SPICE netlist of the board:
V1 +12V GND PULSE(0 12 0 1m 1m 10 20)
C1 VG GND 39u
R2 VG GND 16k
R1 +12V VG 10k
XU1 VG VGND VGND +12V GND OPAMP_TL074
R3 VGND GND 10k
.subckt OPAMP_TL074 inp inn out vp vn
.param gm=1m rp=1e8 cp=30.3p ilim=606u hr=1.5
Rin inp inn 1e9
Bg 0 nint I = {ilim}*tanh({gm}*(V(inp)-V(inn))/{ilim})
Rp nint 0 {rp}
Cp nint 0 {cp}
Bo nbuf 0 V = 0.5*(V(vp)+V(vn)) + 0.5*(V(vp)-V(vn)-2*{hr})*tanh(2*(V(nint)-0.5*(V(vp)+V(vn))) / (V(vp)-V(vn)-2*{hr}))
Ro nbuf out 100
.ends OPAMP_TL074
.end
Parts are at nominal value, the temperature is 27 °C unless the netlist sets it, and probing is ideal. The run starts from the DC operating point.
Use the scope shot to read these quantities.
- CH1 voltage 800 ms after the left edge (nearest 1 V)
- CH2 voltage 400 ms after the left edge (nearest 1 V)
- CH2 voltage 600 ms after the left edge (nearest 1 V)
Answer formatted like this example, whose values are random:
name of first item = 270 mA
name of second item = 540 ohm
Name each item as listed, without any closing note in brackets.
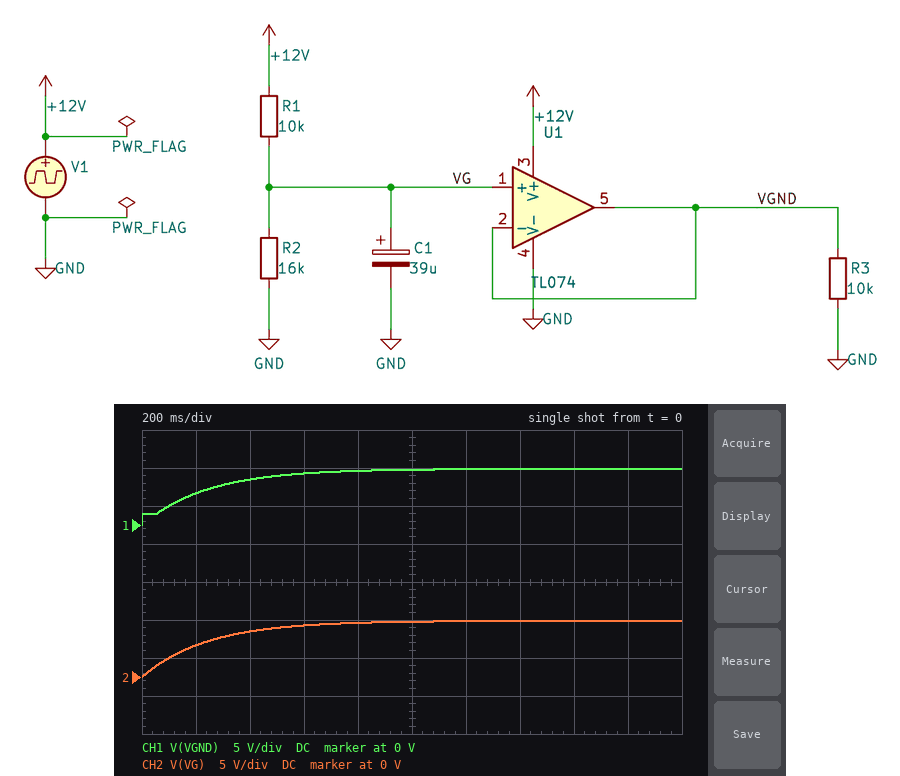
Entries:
CH1 voltage 800 ms after the left edge = 7 V
CH2 voltage 400 ms after the left edge = 6 V
CH2 voltage 600 ms after the left edge = 7 V
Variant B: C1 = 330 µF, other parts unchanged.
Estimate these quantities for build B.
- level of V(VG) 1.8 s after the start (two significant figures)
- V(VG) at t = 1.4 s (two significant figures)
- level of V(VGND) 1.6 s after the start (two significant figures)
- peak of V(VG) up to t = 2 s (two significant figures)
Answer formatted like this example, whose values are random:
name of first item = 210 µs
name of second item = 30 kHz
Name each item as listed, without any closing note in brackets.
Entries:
level of V(VG) 1.8 s after the start = 4.3 V
V(VG) at t = 1.4 s = 3.7 V
level of V(VGND) 1.6 s after the start = 4.0 V
peak of V(VG) up to t = 2 s = 4.6 V
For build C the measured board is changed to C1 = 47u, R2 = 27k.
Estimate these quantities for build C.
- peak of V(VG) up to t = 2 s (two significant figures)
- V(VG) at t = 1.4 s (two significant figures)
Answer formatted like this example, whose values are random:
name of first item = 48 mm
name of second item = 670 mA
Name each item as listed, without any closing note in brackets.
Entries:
peak of V(VG) up to t = 2 s = 8.7 V
V(VG) at t = 1.4 s = 8.6 V
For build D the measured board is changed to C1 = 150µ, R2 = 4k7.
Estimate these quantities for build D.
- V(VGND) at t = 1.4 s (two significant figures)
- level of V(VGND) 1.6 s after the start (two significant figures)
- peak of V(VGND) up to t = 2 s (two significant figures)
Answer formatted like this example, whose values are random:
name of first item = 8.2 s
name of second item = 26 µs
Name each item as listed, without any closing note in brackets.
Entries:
V(VGND) at t = 1.4 s = 3.6 V
level of V(VGND) 1.6 s after the start = 3.7 V
peak of V(VGND) up to t = 2 s = 3.8 V
